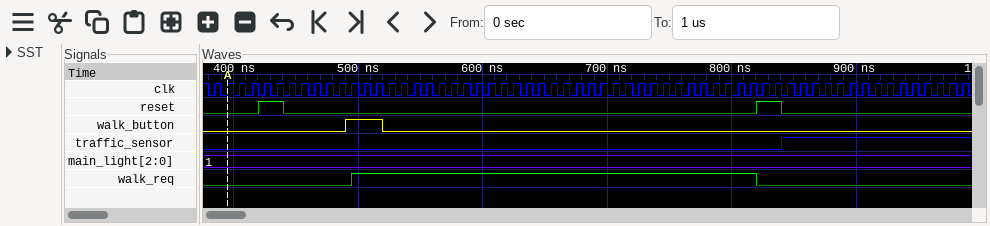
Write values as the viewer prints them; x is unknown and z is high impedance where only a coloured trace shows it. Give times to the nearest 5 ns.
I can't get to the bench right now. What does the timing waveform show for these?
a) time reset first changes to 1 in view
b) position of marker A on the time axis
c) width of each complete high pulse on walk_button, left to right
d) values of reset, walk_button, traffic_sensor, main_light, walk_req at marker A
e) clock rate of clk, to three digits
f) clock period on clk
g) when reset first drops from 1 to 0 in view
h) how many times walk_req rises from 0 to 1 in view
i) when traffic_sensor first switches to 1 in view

420 ns
395 ns
30 ns
reset=0, walk_button=0, traffic_sensor=0, main_light=1, walk_req=0
100 MHz
10 ns
440 ns
1
840 ns
